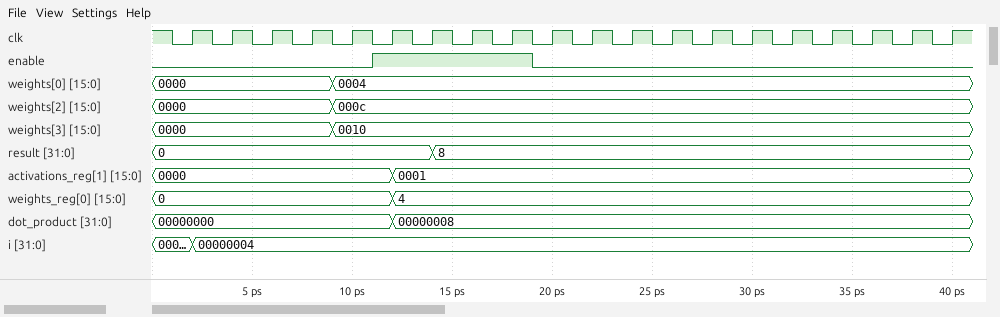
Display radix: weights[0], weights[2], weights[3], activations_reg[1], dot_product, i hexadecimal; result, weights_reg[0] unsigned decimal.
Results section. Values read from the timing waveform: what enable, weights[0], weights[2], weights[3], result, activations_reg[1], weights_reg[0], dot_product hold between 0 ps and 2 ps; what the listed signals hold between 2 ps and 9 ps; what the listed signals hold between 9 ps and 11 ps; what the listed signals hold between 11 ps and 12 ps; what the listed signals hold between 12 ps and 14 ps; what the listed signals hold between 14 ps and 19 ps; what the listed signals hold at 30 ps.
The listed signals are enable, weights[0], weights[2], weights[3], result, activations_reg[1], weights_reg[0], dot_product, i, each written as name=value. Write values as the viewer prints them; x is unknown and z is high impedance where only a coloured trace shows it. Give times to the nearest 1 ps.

enable=0, weights[0]=0000, weights[2]=0000, weights[3]=0000, result=0, activations_reg[1]=0000, weights_reg[0]=0, dot_product=00000000
enable=0, weights[0]=0000, weights[2]=0000, weights[3]=0000, result=0, activations_reg[1]=0000, weights_reg[0]=0, dot_product=00000000, i=00000004
enable=0, weights[0]=0004, weights[2]=000c, weights[3]=0010, result=0, activations_reg[1]=0000, weights_reg[0]=0, dot_product=00000000, i=00000004
enable=1, weights[0]=0004, weights[2]=000c, weights[3]=0010, result=0, activations_reg[1]=0000, weights_reg[0]=0, dot_product=00000000, i=00000004
enable=1, weights[0]=0004, weights[2]=000c, weights[3]=0010, result=0, activations_reg[1]=0001, weights_reg[0]=4, dot_product=00000008, i=00000004
enable=1, weights[0]=0004, weights[2]=000c, weights[3]=0010, result=8, activations_reg[1]=0001, weights_reg[0]=4, dot_product=00000008, i=00000004
enable=0, weights[0]=0004, weights[2]=000c, weights[3]=0010, result=8, activations_reg[1]=0001, weights_reg[0]=4, dot_product=00000008, i=00000004
